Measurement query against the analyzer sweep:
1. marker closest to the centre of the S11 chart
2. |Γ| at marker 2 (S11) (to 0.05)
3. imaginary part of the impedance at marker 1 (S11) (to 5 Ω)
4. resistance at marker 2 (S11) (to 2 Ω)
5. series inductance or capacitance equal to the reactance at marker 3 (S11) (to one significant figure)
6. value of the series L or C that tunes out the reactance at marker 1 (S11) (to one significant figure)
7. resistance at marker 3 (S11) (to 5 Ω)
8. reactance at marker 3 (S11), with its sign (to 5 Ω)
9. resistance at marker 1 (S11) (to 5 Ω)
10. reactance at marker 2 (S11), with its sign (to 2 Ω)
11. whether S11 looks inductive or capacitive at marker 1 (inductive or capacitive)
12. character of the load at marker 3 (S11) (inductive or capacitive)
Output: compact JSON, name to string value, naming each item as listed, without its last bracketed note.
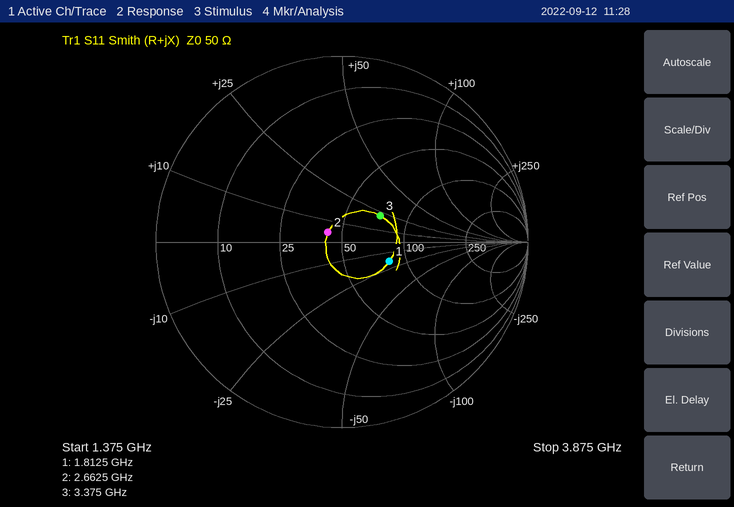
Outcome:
{"marker closest to the centre of the S11 chart": "marker 2", "|Γ| at marker 2 (S11)": "0.10", "imaginary part of the impedance at marker 1 (S11)": "-20 Ω", "resistance at marker 2 (S11)": "42 Ω", "series inductance or capacitance equal to the reactance at marker 3 (S11)": "1 nH", "value of the series L or C that tunes out the reactance at marker 1 (S11)": "2 nH", "resistance at marker 3 (S11)": "70 Ω", "reactance at marker 3 (S11), with its sign": "+20 Ω", "resistance at marker 1 (S11)": "80 Ω", "reactance at marker 2 (S11), with its sign": "+4 Ω", "whether S11 looks inductive or capacitive at marker 1": "capacitive", "character of the load at marker 3 (S11)": "inductive"}
